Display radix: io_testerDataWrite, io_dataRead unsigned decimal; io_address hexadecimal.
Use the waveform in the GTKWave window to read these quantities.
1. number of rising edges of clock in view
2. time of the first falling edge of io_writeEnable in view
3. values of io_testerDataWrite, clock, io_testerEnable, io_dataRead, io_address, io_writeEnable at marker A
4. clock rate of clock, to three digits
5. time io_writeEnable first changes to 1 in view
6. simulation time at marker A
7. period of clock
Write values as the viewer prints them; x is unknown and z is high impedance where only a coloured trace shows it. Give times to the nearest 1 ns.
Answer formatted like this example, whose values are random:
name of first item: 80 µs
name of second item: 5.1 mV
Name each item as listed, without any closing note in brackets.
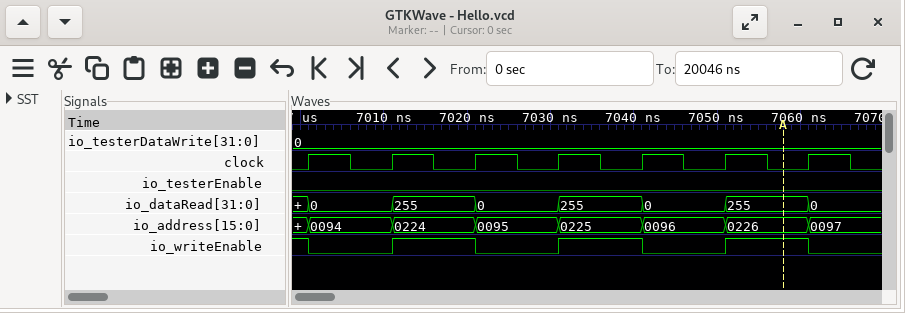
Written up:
number of rising edges of clock in view: 7
time of the first falling edge of io_writeEnable in view: 7001 ns
values of io_testerDataWrite, clock, io_testerEnable, io_dataRead, io_address, io_writeEnable at marker A: io_testerDataWrite=0, clock=0, io_testerEnable=0, io_dataRead=255, io_address=0226, io_writeEnable=1
clock rate of clock, to three digits: 100 MHz
time io_writeEnable first changes to 1 in view: 7011 ns
simulation time at marker A: 7058 ns
period of clock: 10 ns
